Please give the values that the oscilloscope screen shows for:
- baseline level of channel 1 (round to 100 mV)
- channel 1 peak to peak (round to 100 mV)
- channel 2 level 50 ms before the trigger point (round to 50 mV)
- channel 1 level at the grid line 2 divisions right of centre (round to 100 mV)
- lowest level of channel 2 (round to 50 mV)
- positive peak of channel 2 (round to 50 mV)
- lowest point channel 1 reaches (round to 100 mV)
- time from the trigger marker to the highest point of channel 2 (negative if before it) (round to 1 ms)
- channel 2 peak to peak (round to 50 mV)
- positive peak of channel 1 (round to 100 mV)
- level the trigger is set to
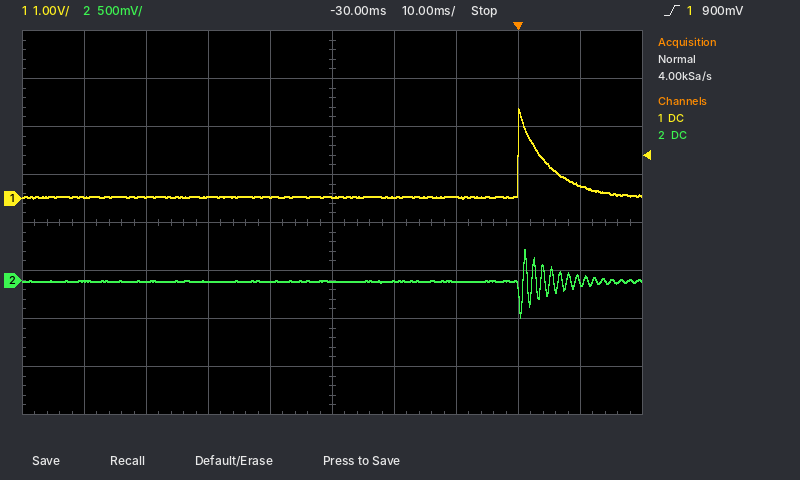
0.0 V
1.9 V
0 mV
0.0 V
-400 mV
300 mV
0.0 V
+1 ms
700 mV
1.9 V
900 mV
